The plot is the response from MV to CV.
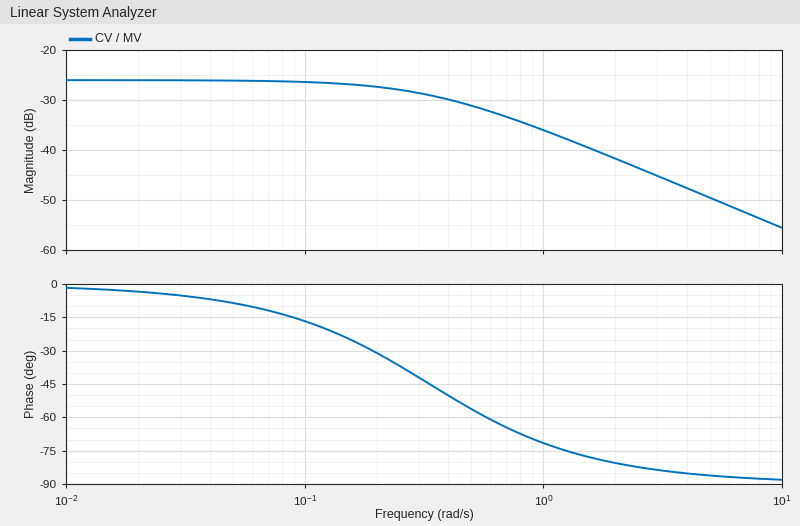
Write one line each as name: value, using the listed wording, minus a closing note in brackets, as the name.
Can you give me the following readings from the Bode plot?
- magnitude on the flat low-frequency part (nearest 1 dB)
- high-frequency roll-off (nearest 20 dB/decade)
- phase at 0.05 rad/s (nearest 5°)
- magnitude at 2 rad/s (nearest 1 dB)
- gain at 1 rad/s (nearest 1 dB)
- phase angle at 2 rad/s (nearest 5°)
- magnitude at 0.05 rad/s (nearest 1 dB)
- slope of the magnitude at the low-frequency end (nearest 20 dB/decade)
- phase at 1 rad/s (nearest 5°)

magnitude on the flat low-frequency part: -26 dB
high-frequency roll-off: -20 dB/decade
phase at 0.05 rad/s: -10°
magnitude at 2 rad/s: -42 dB
gain at 1 rad/s: -36 dB
phase angle at 2 rad/s: -80°
magnitude at 0.05 rad/s: -26 dB
slope of the magnitude at the low-frequency end: 0 dB/decade
phase at 1 rad/s: -70°
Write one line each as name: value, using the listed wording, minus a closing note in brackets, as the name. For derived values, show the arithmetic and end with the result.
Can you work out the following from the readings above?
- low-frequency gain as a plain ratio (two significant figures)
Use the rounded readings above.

low-frequency gain as a plain ratio: 10^(-26 / 20) = 0.050
